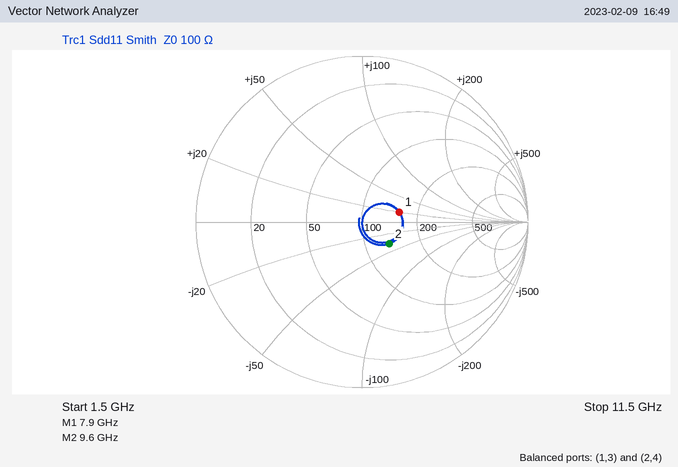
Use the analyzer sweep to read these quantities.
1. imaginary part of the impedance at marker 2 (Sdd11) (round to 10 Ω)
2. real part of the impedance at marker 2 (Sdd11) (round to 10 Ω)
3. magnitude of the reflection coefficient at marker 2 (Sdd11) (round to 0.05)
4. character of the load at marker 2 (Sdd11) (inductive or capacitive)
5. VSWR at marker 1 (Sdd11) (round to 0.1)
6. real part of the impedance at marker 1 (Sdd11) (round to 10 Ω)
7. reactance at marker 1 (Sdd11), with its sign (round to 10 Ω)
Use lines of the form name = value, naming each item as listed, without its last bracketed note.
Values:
imaginary part of the impedance at marker 2 (Sdd11) = -40 Ω
real part of the impedance at marker 2 (Sdd11) = 130 Ω
magnitude of the reflection coefficient at marker 2 (Sdd11) = 0.20
character of the load at marker 2 (Sdd11) = capacitive
VSWR at marker 1 (Sdd11) = 1.6
real part of the impedance at marker 1 (Sdd11) = 160 Ω
reactance at marker 1 (Sdd11), with its sign = +20 Ω
